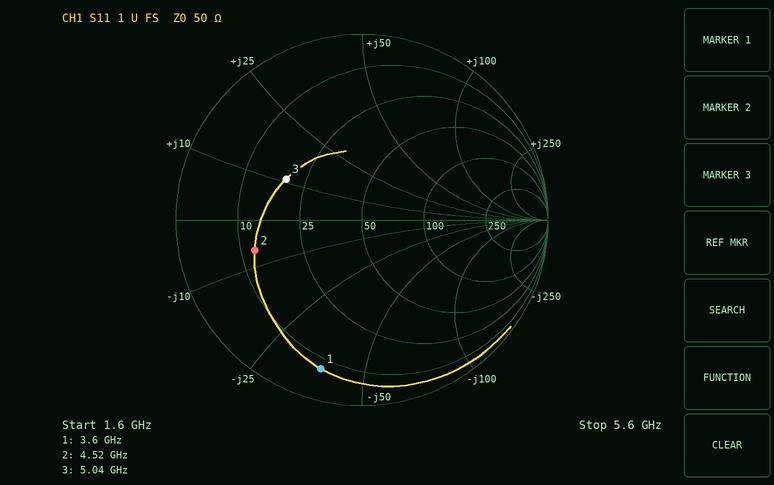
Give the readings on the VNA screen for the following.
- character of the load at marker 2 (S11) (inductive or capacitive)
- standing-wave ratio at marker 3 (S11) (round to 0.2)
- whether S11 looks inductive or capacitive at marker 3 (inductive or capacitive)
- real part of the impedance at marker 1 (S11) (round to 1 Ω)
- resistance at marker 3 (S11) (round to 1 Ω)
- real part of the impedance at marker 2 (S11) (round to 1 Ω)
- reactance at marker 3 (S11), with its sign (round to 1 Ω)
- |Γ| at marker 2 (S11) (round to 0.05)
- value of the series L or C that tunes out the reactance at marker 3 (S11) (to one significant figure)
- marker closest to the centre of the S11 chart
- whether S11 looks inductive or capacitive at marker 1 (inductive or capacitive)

capacitive
2.8
inductive
7 Ω
19 Ω
13 Ω
+11 Ω
0.60
3 pF
marker 3
capacitive
